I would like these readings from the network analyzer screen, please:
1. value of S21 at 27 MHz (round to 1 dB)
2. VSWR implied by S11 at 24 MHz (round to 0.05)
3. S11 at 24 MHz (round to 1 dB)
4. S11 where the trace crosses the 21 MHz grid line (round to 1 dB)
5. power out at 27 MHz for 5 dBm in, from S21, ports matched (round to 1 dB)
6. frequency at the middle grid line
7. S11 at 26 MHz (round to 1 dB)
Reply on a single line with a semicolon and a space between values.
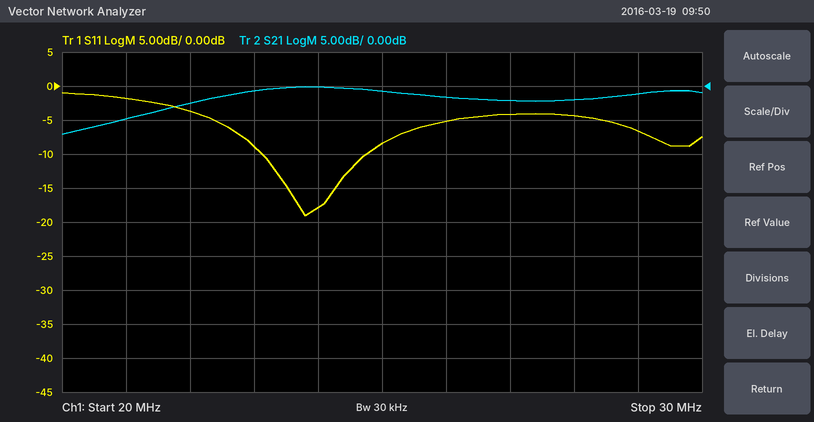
-2 dB; 1.30; -18 dB; -2 dB; 3 dBm; 25 MHz; -5 dB
